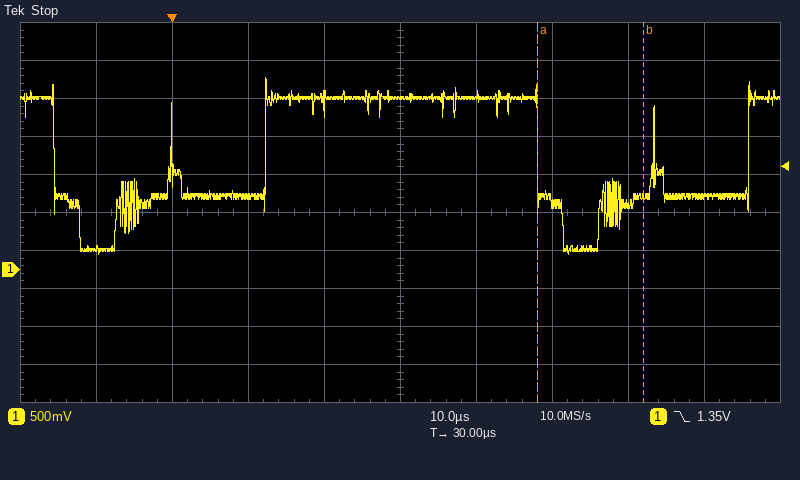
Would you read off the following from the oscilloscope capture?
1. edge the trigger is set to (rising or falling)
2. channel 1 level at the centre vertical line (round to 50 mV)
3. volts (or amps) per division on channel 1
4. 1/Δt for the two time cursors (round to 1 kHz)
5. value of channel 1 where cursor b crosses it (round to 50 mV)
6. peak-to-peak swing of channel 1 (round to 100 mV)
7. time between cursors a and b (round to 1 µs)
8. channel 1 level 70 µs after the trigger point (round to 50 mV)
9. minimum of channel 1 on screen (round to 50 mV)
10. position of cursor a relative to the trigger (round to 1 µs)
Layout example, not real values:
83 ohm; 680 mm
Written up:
falling; 2.25 V; 500 mV; 71 kHz; 950 mV; 2.30 V; 14 µs; 950 mV; 200 mV; +48 µs
